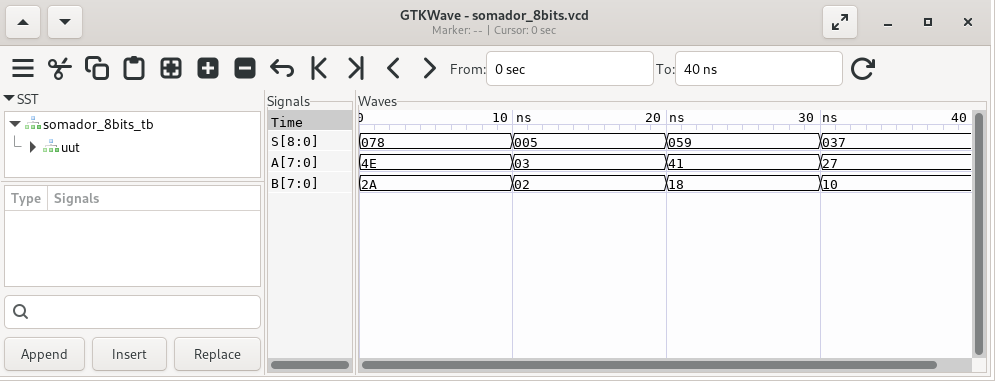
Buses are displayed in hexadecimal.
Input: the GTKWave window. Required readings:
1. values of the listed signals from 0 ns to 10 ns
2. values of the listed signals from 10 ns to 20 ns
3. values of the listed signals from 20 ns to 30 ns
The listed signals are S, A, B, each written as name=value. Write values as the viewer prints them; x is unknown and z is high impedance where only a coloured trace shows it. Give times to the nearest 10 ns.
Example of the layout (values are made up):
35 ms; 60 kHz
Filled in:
S=078, A=4E, B=2A; S=005, A=03, B=02; S=059, A=41, B=18
